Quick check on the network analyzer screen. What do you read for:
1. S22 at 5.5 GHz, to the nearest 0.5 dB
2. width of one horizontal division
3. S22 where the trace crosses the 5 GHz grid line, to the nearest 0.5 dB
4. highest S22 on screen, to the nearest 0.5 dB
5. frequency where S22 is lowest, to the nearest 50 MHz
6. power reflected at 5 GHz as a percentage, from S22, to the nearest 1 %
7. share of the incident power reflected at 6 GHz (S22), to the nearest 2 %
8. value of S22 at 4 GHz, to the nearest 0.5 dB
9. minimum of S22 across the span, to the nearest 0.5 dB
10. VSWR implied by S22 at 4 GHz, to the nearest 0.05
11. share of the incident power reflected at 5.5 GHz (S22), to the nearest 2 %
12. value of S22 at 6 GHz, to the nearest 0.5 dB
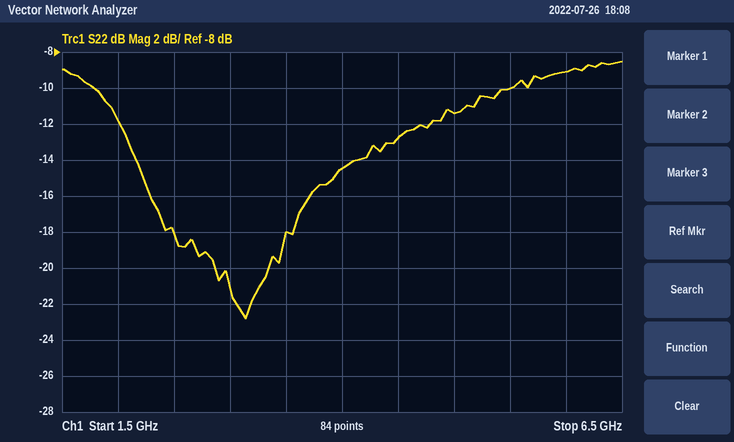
-10.0 dB
500 MHz
-11.5 dB
-8.5 dB
3.15 GHz
7 %
12 %
-14.5 dB
-23.0 dB
1.45
10 %
-9.0 dB
